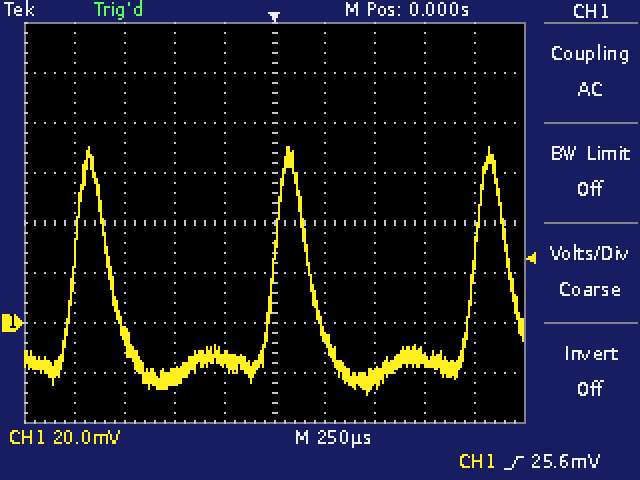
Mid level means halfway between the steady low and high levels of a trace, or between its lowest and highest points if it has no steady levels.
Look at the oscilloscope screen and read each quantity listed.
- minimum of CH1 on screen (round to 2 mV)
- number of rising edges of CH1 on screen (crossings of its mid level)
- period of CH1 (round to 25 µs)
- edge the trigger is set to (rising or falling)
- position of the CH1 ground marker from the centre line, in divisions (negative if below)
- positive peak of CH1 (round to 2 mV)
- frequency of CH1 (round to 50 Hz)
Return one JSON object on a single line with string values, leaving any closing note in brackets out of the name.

{"minimum of CH1 on screen": "-28 mV", "number of rising edges of CH1 on screen": "3", "period of CH1": "1.000 ms", "edge the trigger is set to": "rising", "position of the CH1 ground marker from the centre line, in divisions": "-2.0 div", "positive peak of CH1": "70 mV", "frequency of CH1": "1.00 kHz"}
